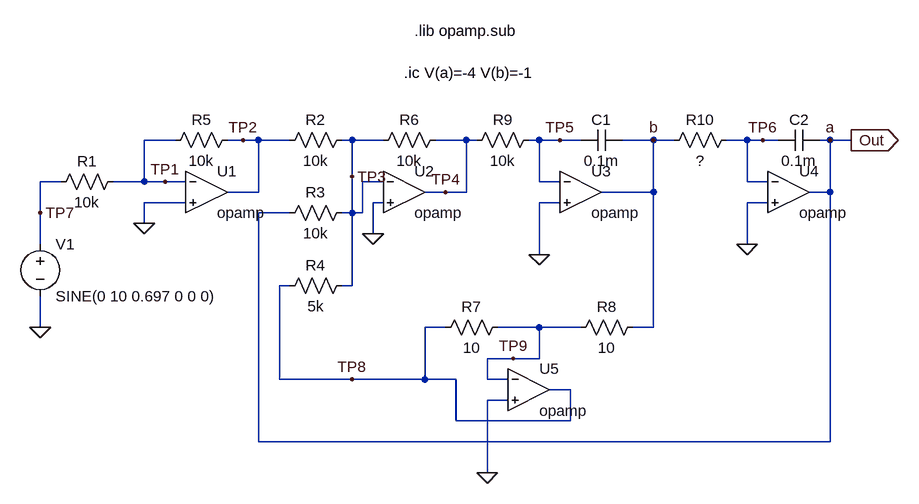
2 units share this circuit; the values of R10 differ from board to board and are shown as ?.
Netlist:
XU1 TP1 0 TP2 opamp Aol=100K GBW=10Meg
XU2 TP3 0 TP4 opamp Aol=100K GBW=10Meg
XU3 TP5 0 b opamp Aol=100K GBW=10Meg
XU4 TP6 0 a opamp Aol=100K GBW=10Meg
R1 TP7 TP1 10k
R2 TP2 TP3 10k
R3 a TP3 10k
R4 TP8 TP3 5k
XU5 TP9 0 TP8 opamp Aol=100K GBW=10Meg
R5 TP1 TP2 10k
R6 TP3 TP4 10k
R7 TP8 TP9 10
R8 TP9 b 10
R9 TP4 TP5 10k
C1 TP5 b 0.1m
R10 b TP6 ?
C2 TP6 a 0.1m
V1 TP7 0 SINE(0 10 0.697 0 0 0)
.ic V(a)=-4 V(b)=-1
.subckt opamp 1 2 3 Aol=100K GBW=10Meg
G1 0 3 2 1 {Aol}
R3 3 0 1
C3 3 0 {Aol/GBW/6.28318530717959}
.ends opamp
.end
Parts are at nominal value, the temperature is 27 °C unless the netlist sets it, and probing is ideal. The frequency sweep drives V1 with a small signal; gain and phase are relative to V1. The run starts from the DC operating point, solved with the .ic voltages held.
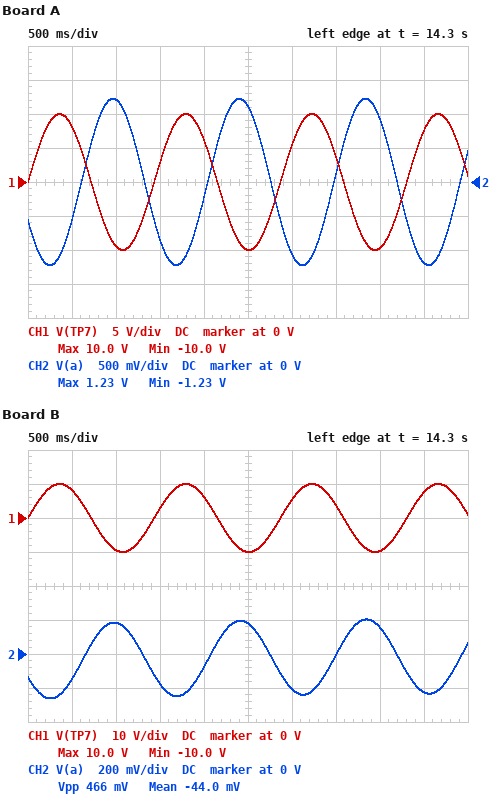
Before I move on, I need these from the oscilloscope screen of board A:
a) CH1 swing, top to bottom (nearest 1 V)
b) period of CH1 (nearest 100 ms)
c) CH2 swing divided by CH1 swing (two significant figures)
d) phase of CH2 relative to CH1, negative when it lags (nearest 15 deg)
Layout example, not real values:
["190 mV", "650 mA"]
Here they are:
["20 V", "1.4 s", "0.12", "-150 deg"]
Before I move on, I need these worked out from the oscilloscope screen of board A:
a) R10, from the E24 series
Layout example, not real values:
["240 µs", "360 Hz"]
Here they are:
["4.3 kΩ"]
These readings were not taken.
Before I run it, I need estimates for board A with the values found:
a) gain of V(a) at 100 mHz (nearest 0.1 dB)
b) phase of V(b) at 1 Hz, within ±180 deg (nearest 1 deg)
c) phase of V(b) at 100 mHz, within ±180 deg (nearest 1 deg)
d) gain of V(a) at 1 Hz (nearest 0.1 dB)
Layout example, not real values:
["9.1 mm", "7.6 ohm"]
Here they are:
["0.1 dB", "109 deg", "-123 deg", "-24.5 dB"]
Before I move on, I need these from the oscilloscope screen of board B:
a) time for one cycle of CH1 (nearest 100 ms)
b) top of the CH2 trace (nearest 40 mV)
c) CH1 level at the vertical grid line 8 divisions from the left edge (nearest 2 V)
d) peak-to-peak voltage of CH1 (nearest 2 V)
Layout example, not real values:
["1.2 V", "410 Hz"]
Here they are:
["1.4 s", "200 mV", "-10 V", "20 V"]
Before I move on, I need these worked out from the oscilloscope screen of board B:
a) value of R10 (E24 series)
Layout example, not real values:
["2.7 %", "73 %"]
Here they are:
["22 kΩ"]
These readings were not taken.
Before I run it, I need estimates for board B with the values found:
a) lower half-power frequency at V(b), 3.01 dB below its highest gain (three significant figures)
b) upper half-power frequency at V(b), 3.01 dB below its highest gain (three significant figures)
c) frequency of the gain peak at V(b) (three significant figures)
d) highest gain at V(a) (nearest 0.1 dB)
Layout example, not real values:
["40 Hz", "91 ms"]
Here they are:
["32.8 mHz", "351 mHz", "107 mHz", "0 dB"]
